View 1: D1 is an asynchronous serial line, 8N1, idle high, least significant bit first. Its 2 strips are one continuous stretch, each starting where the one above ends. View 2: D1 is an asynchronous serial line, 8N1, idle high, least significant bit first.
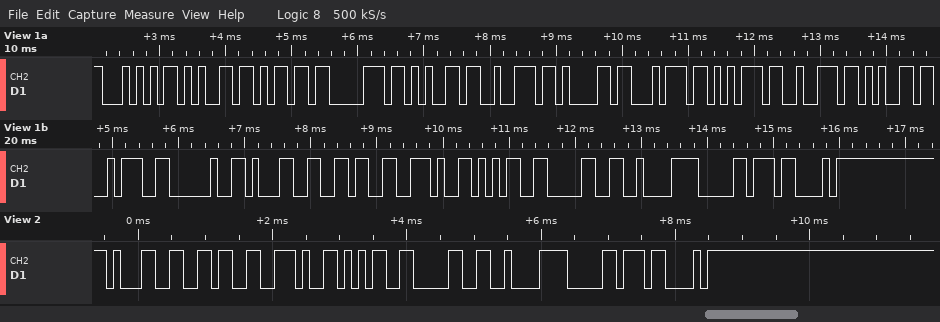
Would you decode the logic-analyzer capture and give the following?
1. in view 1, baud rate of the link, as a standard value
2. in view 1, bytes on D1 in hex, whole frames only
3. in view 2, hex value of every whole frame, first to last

9600 baud
54 65 6D 70 65 72 61 74 75 72 65 3A 20 31 36 2E 35 30 C2 B0 43
31 36 2E 35 30 C2 B0 43
